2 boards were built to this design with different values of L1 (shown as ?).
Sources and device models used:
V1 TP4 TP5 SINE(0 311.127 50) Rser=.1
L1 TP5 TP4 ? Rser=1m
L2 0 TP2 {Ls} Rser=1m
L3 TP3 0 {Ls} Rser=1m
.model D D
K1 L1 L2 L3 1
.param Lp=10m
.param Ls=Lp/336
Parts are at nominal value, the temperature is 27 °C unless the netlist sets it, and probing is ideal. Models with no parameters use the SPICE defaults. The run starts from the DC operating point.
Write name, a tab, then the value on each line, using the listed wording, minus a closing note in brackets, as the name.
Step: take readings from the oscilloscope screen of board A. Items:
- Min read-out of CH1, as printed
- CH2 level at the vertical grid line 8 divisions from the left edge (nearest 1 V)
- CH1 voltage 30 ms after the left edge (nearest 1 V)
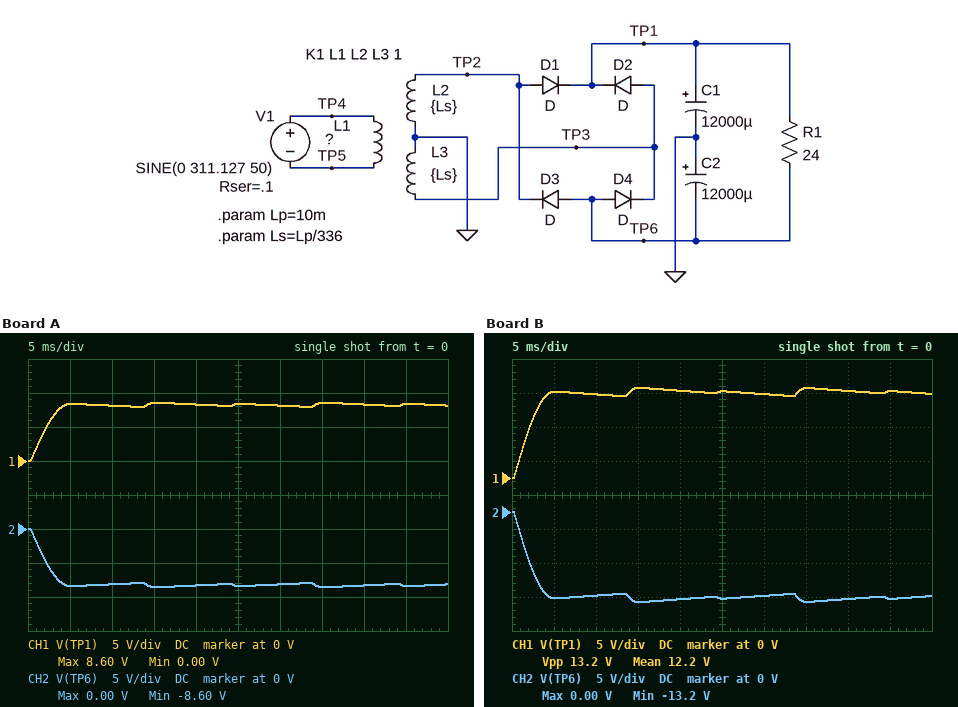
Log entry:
Min read-out of CH1, as printed	0.00 V
CH2 level at the vertical grid line 8 divisions from the left edge	-8 V
CH1 voltage 30 ms after the left edge	8 V
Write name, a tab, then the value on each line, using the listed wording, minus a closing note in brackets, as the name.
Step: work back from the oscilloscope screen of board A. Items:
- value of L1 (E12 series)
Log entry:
value of L1	33 mH
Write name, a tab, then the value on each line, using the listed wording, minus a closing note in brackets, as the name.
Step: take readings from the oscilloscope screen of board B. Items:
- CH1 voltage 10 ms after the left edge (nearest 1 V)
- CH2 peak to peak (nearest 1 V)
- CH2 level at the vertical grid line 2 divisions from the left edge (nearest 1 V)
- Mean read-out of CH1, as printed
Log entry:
CH1 voltage 10 ms after the left edge	12 V
CH2 peak to peak	13 V
CH2 level at the vertical grid line 2 divisions from the left edge	-12 V
Mean read-out of CH1, as printed	12.2 V
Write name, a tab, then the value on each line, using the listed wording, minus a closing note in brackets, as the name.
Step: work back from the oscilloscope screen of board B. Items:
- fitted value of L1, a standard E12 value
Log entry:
fitted value of L1, a standard E12 value	15 mH
